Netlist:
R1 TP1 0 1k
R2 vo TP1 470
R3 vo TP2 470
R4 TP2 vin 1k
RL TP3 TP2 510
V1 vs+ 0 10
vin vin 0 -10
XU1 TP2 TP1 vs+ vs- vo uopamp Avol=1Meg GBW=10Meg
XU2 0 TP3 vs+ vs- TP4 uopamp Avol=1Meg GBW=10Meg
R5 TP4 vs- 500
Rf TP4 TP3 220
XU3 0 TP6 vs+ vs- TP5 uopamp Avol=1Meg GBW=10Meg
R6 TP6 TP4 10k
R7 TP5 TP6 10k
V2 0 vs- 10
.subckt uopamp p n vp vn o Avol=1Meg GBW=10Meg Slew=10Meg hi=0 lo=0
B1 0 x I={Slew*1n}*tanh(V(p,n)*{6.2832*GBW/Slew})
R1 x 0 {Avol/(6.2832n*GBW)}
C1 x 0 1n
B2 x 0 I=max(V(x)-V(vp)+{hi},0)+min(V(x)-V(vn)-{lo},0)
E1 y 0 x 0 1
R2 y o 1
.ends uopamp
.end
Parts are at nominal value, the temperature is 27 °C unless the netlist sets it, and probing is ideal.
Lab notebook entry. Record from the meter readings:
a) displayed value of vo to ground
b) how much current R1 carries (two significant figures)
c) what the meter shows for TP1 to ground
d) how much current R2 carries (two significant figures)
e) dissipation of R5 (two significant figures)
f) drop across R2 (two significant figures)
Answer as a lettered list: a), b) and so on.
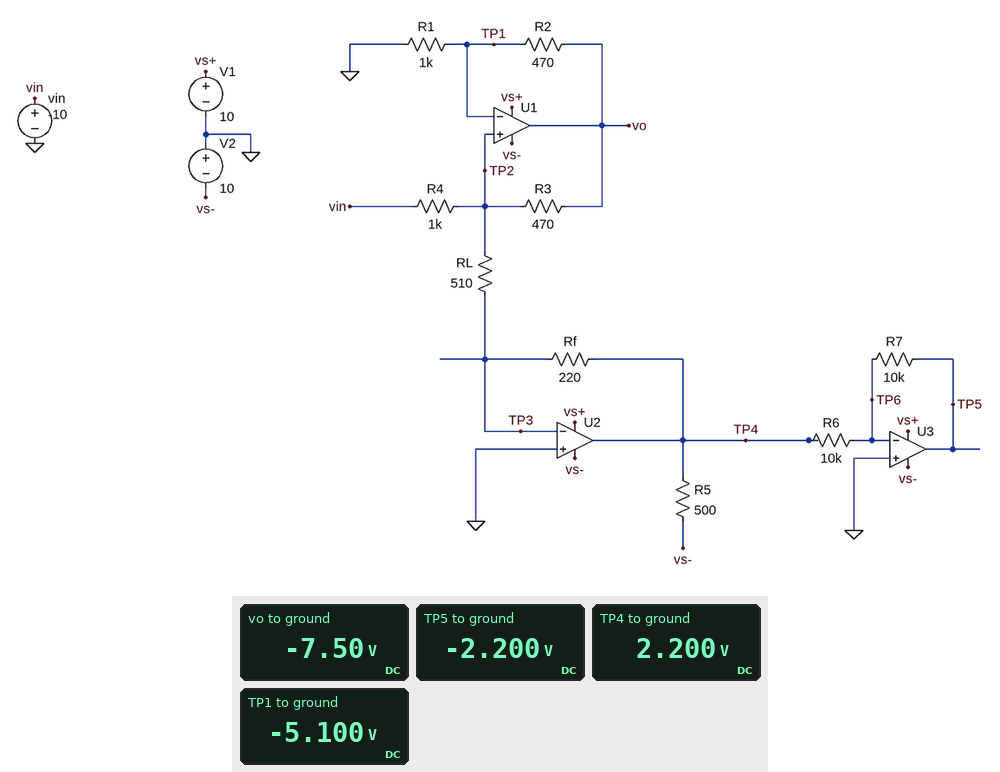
a) -7.50 V
b) 5.1 mA
c) -5.100 V
d) 5.1 mA
e) 300 mW
f) 2.4 V
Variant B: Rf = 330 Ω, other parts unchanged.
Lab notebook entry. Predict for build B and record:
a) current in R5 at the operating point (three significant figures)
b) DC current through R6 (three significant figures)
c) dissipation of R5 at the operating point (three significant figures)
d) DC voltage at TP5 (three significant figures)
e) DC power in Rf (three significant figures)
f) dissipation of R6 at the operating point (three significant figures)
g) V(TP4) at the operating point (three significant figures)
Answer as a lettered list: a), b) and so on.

a) 26.6 mA
b) 330 µA
c) 354 mW
d) -3.30 V
e) 33.0 mW
f) 1.09 mW
g) 3.30 V
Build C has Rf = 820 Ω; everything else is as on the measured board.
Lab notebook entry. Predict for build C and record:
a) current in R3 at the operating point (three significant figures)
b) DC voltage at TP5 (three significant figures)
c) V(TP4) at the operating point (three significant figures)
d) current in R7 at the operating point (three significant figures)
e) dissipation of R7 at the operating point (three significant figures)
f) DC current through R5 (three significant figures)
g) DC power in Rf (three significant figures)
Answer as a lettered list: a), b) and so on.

a) 5.10 mA
b) -8.20 V
c) 8.20 V
d) 820 µA
e) 6.72 mW
f) 36.4 mA
g) 82.0 mW
